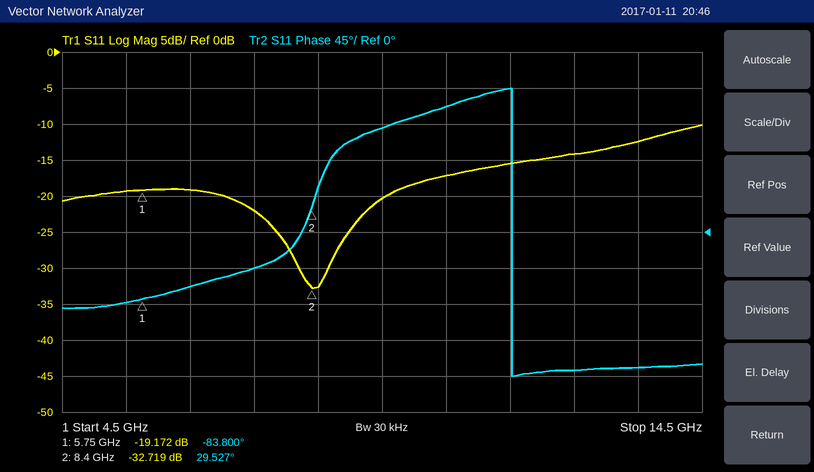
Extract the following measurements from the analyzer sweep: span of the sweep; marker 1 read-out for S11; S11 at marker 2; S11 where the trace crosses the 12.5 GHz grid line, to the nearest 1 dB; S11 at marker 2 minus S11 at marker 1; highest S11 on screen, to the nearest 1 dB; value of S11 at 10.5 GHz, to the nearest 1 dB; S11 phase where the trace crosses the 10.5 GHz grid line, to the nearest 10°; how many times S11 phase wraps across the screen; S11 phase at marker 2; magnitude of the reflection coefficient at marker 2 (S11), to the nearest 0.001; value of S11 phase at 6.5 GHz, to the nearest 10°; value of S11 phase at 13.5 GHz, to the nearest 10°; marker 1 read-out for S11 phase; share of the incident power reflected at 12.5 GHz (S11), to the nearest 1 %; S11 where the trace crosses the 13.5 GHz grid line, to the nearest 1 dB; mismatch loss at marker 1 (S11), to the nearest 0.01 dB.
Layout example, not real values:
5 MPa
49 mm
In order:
10 GHz
-19.172 dB
-32.719 dB
-14 dB
-13.547 dB
-10 dB
-17 dB
160°
1
29.527°
0.023
-70°
-170°
-83.800°
4 %
-12 dB
0.05 dB
